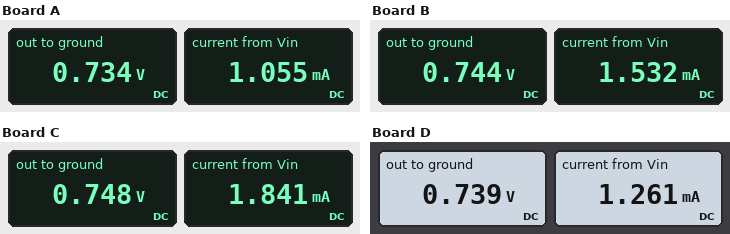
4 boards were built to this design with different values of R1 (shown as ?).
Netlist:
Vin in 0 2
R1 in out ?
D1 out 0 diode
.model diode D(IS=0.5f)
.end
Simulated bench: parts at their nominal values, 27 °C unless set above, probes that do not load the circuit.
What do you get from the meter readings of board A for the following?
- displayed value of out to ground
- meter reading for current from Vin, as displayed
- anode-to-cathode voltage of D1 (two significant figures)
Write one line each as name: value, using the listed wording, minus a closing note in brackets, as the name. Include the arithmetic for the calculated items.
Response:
displayed value of out to ground: 0.734 V
meter reading for current from Vin, as displayed: 1.055 mA
anode-to-cathode voltage of D1: 734 mV = 730 mV
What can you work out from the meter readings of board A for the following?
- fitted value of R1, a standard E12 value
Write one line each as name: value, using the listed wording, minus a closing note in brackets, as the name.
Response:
fitted value of R1, a standard E12 value: 1.2 kΩ
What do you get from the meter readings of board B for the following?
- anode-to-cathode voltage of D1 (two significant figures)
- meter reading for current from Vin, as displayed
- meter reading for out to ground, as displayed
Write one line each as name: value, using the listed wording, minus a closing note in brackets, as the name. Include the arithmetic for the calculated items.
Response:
anode-to-cathode voltage of D1: 744 mV = 740 mV
meter reading for current from Vin, as displayed: 1.532 mA
meter reading for out to ground, as displayed: 0.744 V
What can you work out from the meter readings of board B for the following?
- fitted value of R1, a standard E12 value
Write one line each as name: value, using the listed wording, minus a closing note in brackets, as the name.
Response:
fitted value of R1, a standard E12 value: 820 Ω
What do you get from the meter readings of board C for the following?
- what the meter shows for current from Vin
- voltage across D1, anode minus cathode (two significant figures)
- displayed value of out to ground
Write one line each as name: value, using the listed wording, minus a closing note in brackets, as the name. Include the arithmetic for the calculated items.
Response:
what the meter shows for current from Vin: 1.841 mA
voltage across D1, anode minus cathode: 748 mV = 750 mV
displayed value of out to ground: 0.748 V
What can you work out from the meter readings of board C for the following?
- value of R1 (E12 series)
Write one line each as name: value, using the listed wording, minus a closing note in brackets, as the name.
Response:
value of R1: 680 Ω
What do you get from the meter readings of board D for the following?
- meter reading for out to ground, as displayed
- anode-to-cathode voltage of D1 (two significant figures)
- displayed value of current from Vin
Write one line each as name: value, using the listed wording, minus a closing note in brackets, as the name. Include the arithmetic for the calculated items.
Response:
meter reading for out to ground, as displayed: 0.739 V
anode-to-cathode voltage of D1: 739 mV = 740 mV
displayed value of current from Vin: 1.261 mA
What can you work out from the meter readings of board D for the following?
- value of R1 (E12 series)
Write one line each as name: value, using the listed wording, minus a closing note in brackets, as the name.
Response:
value of R1: 1 kΩ
